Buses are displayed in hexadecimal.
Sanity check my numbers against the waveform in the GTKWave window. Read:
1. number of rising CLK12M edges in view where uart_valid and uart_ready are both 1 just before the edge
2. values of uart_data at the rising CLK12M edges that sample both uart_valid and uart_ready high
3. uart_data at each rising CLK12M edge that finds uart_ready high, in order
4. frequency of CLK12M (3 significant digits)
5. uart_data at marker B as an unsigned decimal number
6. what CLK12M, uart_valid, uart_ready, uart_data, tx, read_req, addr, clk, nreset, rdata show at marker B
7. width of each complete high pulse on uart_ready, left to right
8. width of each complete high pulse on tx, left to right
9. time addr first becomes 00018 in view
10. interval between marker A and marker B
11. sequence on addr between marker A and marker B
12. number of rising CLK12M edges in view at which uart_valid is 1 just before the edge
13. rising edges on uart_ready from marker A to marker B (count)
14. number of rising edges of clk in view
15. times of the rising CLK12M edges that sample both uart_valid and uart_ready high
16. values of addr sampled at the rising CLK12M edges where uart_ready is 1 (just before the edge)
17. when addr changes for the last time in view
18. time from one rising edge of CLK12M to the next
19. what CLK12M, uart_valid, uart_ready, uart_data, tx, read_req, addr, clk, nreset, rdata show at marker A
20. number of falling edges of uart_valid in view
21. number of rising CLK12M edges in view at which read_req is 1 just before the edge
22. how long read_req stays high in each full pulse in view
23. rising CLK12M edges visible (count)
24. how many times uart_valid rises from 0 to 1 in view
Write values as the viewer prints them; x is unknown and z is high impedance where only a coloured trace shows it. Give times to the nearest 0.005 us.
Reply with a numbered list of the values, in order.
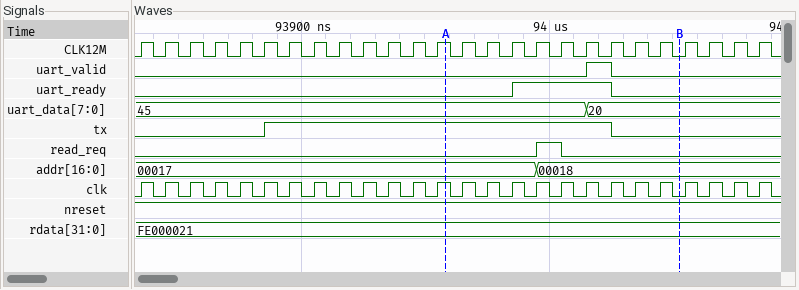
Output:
1. 1
2. 20
3. 45, 45, 45, 20
4. 100 MHz
5. 32
6. CLK12M=0, uart_valid=0, uart_ready=0, uart_data=20, tx=0, read_req=0, addr=00018, clk=0, nreset=1, rdata=FE000021
7. 0.04 us
8. 0.14 us
9. 93.995 us
10. 0.095 us
11. 00017, 00018
12. 1
13. 1
14. 26
15. 94.025 us
16. 00017, 00018, 00018, 00018
17. 93.995 us
18. 0.01 us
19. CLK12M=1, uart_valid=0, uart_ready=0, uart_data=45, tx=1, read_req=0, addr=00017, clk=1, nreset=1, rdata=FE000021
20. 1
21. 1
22. 0.01 us
23. 26
24. 1
